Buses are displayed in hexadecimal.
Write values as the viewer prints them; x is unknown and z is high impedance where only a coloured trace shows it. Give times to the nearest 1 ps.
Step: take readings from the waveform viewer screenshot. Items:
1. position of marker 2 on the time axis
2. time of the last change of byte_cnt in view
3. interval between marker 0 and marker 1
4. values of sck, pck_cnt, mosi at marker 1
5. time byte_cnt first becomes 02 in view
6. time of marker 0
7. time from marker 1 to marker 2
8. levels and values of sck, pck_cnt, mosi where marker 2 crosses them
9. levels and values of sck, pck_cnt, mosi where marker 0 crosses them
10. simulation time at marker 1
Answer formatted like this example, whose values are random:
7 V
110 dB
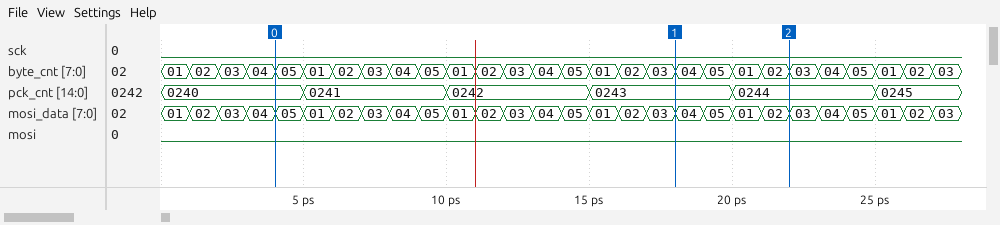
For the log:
22 ps
27 ps
14 ps
sck=0, pck_cnt=0243, mosi=0
1 ps
4 ps
4 ps
sck=0, pck_cnt=0244, mosi=0
sck=0, pck_cnt=0240, mosi=0
18 ps
